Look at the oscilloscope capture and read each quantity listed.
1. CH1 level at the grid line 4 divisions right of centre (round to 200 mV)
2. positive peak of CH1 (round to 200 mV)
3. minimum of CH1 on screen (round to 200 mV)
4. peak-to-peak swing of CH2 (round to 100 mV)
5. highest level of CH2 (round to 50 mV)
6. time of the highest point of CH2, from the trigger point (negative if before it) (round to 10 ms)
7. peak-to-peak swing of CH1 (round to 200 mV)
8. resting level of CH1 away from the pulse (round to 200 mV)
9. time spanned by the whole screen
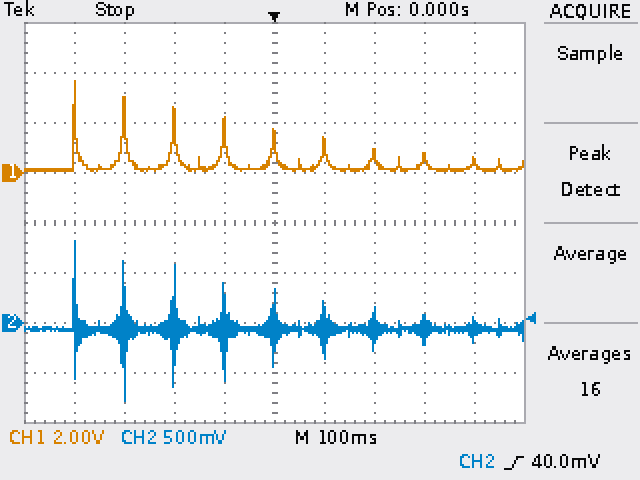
400 mV
3.6 V
0.0 V
1.60 V
800 mV
-400 ms
3.6 V
200 mV
1 s
